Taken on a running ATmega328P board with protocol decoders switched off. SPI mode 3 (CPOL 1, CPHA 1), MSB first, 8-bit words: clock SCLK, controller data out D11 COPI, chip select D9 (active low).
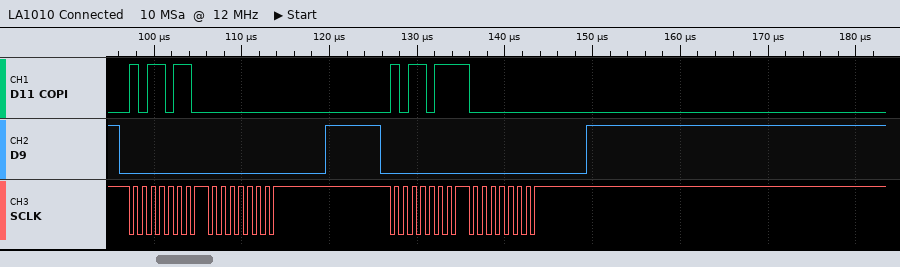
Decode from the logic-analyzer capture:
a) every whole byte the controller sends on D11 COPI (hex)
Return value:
0xB6 0x00 0xB7 0x00
